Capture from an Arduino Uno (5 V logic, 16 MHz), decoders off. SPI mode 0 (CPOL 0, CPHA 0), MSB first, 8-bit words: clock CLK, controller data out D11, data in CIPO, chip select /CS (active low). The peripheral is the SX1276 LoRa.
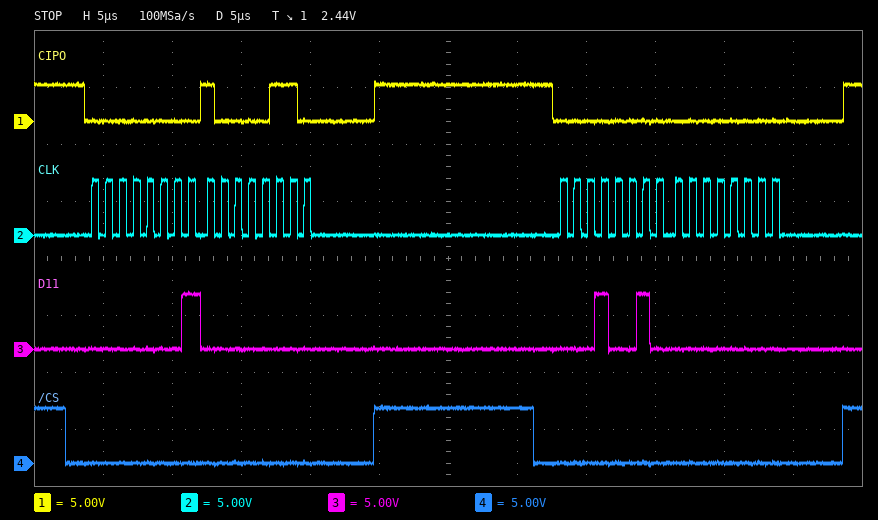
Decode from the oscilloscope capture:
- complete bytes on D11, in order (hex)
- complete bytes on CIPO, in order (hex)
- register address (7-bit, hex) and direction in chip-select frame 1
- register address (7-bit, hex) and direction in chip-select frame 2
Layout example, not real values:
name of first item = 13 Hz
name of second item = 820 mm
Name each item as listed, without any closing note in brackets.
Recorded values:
complete bytes on D11, in order = 0x01 0x00 0x12 0x00
complete bytes on CIPO, in order = 0x00 0x86 0x00 0x00
register address (7-bit, hex) and direction in chip-select frame 1 = 0x01 read
register address (7-bit, hex) and direction in chip-select frame 2 = 0x12 read
